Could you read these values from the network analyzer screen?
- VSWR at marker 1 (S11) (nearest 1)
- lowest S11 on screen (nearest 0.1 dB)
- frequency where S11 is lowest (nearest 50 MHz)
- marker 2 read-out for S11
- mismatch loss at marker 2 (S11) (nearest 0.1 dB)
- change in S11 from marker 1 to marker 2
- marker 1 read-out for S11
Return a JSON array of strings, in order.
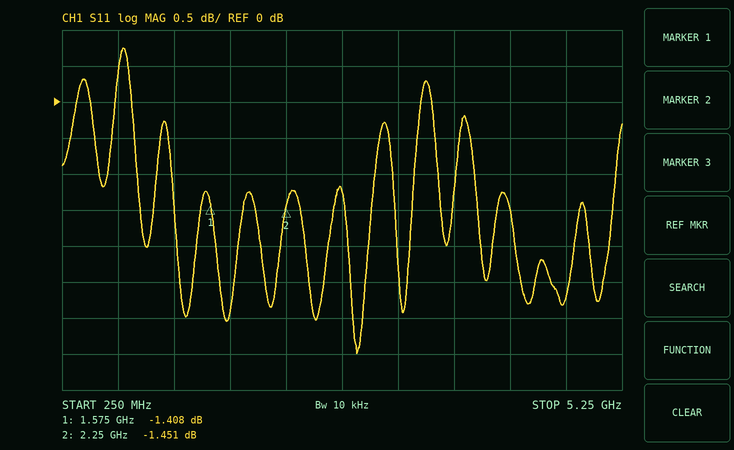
["12", "-3.5 dB", "2.90 GHz", "-1.451 dB", "5.5 dB", "-0.043 dB", "-1.408 dB"]
